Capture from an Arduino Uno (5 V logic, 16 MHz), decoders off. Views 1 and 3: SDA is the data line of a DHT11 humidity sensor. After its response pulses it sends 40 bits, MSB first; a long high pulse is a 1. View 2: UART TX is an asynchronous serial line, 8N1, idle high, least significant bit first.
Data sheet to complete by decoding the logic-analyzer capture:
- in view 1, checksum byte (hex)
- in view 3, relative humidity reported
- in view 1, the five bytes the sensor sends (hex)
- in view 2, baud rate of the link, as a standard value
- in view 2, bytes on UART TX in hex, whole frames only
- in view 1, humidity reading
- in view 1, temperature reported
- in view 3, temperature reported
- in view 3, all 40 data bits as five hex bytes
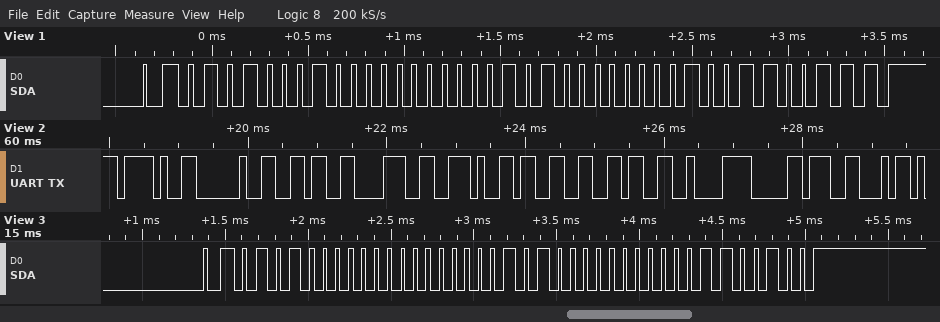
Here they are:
0x67
80 %
51 00 14 02 67
9600 baud
2F 20 36 38 2E 33 36 C2 B0 46
81 %
20.2 °C
20.0 °C
50 00 14 00 64
